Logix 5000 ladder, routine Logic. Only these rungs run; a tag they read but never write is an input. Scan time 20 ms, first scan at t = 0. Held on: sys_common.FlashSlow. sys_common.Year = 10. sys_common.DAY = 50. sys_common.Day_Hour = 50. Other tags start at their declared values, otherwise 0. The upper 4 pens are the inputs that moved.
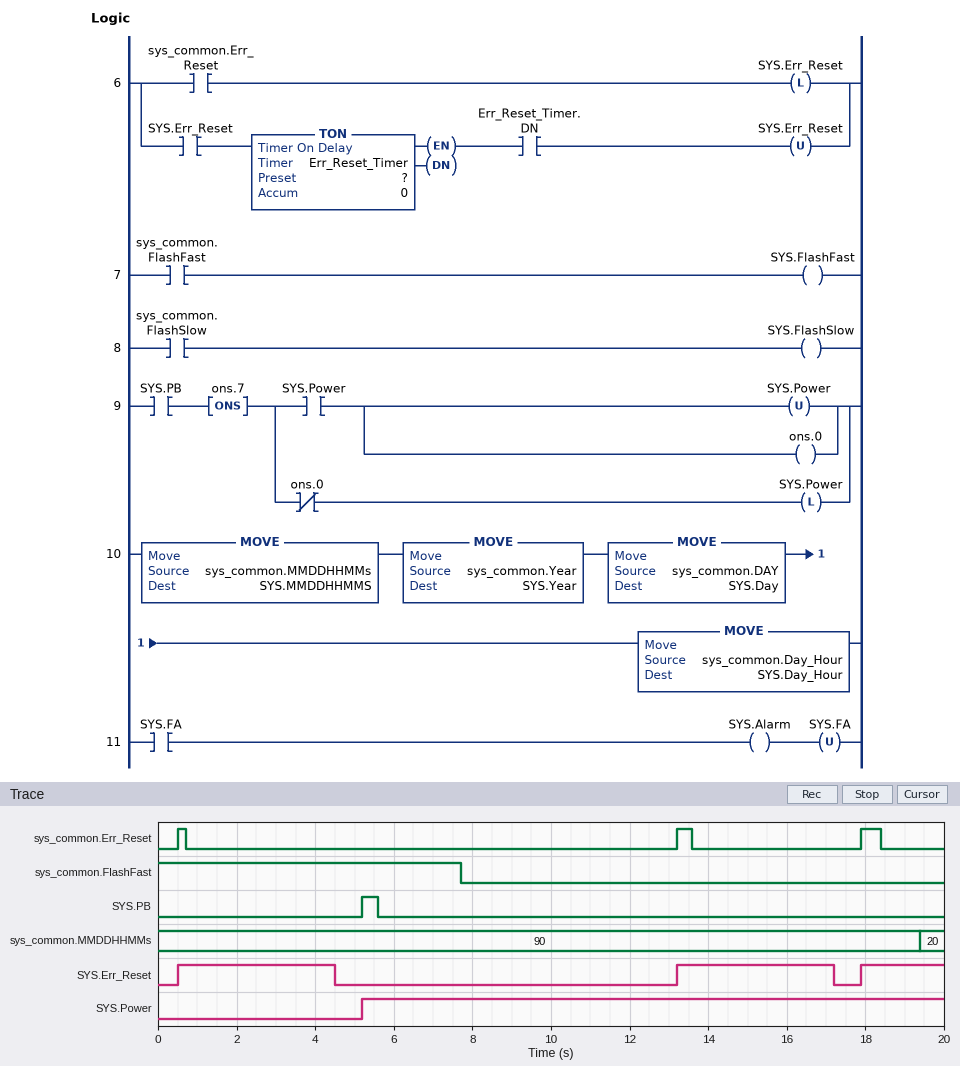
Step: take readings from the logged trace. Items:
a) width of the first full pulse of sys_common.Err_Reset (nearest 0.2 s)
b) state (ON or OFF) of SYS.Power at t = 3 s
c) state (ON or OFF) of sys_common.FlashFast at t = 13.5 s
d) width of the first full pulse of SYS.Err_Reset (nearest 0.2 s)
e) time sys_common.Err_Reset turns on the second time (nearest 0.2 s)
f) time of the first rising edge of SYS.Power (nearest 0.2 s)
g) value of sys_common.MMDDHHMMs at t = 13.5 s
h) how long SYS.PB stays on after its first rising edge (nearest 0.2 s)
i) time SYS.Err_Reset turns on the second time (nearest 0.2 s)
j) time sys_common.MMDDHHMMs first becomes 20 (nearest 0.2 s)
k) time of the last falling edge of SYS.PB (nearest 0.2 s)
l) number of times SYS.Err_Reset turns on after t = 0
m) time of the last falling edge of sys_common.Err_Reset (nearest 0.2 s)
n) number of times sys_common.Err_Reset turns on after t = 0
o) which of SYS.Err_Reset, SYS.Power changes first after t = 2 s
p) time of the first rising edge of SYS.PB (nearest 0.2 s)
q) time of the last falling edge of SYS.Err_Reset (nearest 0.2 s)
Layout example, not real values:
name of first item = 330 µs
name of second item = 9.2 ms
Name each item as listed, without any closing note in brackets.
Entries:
width of the first full pulse of sys_common.Err_Reset = 0.2 s
state (ON or OFF) of SYS.Power at t = 3 s = OFF
state (ON or OFF) of sys_common.FlashFast at t = 13.5 s = OFF
width of the first full pulse of SYS.Err_Reset = 4.0 s
time sys_common.Err_Reset turns on the second time = 13.2 s
time of the first rising edge of SYS.Power = 5.2 s
value of sys_common.MMDDHHMMs at t = 13.5 s = 90
how long SYS.PB stays on after its first rising edge = 0.4 s
time SYS.Err_Reset turns on the second time = 13.2 s
time sys_common.MMDDHHMMs first becomes 20 = 19.4 s
time of the last falling edge of SYS.PB = 5.6 s
number of times SYS.Err_Reset turns on after t = 0 = 3
time of the last falling edge of sys_common.Err_Reset = 18.4 s
number of times sys_common.Err_Reset turns on after t = 0 = 3
which of SYS.Err_Reset, SYS.Power changes first after t = 2 s = SYS.Err_Reset
time of the first rising edge of SYS.PB = 5.2 s
time of the last falling edge of SYS.Err_Reset = 17.2 s
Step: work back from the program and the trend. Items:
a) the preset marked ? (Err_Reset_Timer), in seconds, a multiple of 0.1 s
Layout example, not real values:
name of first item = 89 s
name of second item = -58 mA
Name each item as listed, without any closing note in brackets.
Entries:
the preset marked ? (Err_Reset_Timer), in seconds, a multiple of 0.1 s = 4.0 s
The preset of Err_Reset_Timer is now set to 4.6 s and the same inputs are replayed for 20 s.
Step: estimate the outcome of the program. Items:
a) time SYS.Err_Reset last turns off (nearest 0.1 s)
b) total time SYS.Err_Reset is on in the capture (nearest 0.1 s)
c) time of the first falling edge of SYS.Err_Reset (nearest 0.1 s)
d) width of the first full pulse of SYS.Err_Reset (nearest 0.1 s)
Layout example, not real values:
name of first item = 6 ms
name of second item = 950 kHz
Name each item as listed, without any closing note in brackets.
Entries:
time SYS.Err_Reset last turns off = 17.8 s
total time SYS.Err_Reset is on in the capture = 11.3 s
time of the first falling edge of SYS.Err_Reset = 5.1 s
width of the first full pulse of SYS.Err_Reset = 4.6 s
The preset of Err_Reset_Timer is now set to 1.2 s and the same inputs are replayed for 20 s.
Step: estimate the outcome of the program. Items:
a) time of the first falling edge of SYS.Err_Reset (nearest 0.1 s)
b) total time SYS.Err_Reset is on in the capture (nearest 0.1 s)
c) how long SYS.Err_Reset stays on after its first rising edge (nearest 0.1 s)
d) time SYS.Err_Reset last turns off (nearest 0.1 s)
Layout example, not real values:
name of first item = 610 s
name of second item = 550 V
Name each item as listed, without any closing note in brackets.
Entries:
time of the first falling edge of SYS.Err_Reset = 1.7 s
total time SYS.Err_Reset is on in the capture = 3.6 s
how long SYS.Err_Reset stays on after its first rising edge = 1.2 s
time SYS.Err_Reset last turns off = 19.1 s
